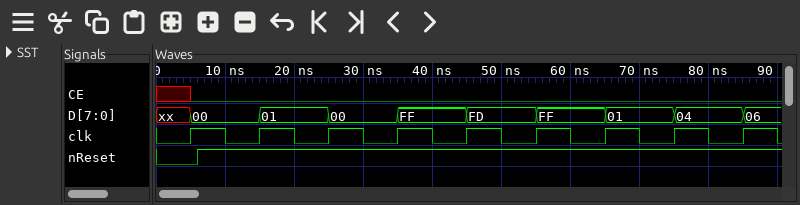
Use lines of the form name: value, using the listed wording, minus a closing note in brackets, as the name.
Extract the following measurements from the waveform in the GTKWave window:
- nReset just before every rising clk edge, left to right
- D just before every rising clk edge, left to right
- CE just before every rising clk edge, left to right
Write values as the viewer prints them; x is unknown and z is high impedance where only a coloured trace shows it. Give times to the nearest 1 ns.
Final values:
nReset just before every rising clk edge, left to right: 0 1 1 1 1 1 1 1 1
D just before every rising clk edge, left to right: xx, 00, 01, 00, FF, FD, FF, 01, 04
CE just before every rising clk edge, left to right: x 0 0 0 0 0 0 0 0
